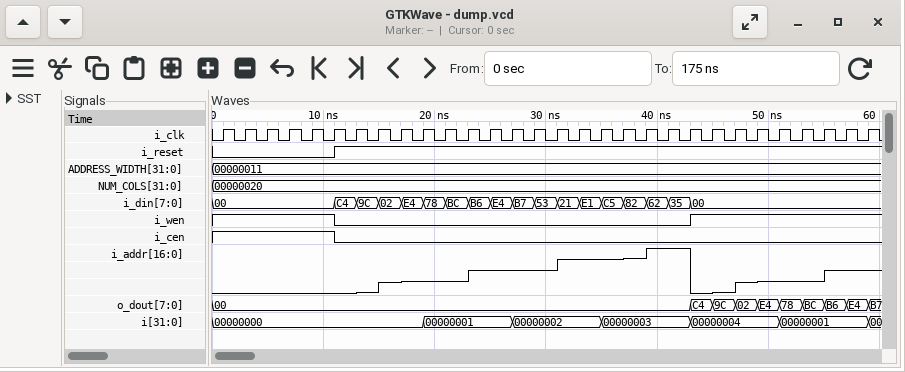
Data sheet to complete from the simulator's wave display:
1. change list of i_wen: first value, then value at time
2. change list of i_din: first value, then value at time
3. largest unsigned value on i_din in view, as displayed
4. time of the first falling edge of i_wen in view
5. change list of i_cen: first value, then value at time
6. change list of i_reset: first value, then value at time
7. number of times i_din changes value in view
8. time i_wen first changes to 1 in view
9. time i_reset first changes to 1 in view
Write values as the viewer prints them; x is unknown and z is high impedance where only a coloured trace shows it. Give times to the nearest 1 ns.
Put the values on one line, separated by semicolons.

1, 0 at 11 ns, 1 at 43 ns; 00, C4 at 11 ns, 9C at 13 ns, 02 at 15 ns, E4 at 17 ns, 78 at 19 ns, BC at 21 ns, B6 at 23 ns, E4 at 25 ns, B7 at 27 ns, 53 at 29 ns, 21 at 31 ns, E1 at 33 ns, C5 at 35 ns, 82 at 37 ns, 62 at 39 ns, 35 at 41 ns, 00 at 43 ns; E4; 11 ns; 1, 0 at 11 ns; 0, 1 at 11 ns; 17; 43 ns; 11 ns
